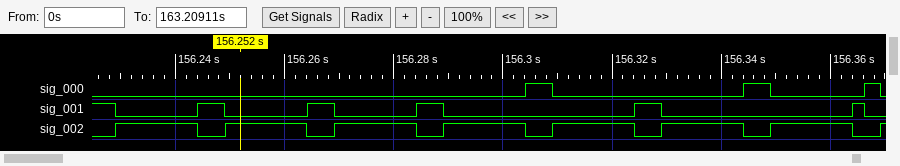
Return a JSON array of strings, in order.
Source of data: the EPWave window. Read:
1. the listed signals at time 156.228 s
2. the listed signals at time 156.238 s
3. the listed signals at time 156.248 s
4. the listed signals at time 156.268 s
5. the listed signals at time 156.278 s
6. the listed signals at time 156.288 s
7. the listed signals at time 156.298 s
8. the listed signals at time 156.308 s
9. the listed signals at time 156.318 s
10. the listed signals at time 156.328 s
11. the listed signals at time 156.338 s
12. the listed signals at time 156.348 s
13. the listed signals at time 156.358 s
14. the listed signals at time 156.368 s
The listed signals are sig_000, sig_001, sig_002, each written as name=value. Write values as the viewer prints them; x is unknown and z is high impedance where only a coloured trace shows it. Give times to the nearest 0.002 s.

["sig_000=0, sig_001=1, sig_002=0", "sig_000=0, sig_001=0, sig_002=1", "sig_000=0, sig_001=1, sig_002=0", "sig_000=0, sig_001=1, sig_002=0", "sig_000=0, sig_001=0, sig_002=1", "sig_000=0, sig_001=1, sig_002=0", "sig_000=0, sig_001=0, sig_002=1", "sig_000=1, sig_001=0, sig_002=0", "sig_000=0, sig_001=0, sig_002=1", "sig_000=0, sig_001=1, sig_002=0", "sig_000=0, sig_001=0, sig_002=1", "sig_000=1, sig_001=0, sig_002=0", "sig_000=0, sig_001=0, sig_002=1", "sig_000=1, sig_001=0, sig_002=0"]
